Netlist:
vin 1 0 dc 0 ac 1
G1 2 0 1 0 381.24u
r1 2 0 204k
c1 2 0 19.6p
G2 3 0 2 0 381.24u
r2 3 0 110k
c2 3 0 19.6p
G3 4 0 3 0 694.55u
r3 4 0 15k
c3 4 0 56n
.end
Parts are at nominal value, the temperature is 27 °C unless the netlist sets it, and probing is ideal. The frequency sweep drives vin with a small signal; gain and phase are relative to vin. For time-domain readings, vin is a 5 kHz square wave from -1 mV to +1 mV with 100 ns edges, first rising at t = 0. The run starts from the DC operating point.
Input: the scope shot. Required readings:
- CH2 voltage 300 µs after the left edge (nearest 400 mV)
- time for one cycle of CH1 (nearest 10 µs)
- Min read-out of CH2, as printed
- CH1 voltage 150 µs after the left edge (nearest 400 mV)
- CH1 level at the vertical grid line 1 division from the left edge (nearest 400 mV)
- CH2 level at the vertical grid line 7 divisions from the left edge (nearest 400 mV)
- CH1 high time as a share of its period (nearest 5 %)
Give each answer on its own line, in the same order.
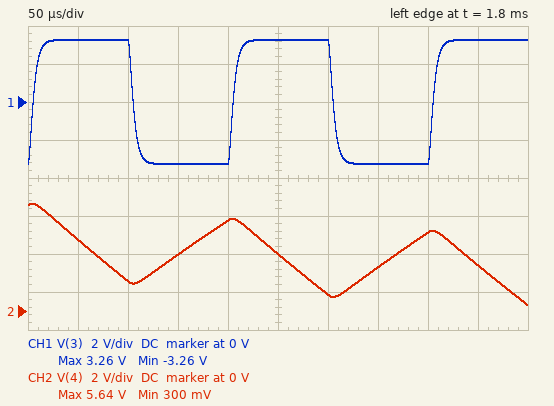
800 mV
200 µs
300 mV
-3.2 V
3.2 V
2.4 V
50 %
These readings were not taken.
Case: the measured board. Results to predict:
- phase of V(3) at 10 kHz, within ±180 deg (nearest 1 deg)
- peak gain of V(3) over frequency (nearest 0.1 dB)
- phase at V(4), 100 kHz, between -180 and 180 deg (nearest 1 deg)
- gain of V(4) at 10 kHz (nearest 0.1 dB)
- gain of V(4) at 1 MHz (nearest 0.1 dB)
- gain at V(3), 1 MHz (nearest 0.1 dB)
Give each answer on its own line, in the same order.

-22 deg
70.3 dB
-32 deg
55.8 dB
-34.5 dB
19.6 dB
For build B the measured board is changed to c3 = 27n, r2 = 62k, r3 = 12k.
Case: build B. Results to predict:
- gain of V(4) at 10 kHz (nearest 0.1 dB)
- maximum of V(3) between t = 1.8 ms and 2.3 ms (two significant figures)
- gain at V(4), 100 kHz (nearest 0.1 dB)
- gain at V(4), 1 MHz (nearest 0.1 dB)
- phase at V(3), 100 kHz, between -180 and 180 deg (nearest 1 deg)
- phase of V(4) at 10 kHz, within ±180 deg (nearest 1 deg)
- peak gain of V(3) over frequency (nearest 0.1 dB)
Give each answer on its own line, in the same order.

57.2 dB
1.8 V
26.9 dB
-28.2 dB
-106 deg
74 deg
65.3 dB
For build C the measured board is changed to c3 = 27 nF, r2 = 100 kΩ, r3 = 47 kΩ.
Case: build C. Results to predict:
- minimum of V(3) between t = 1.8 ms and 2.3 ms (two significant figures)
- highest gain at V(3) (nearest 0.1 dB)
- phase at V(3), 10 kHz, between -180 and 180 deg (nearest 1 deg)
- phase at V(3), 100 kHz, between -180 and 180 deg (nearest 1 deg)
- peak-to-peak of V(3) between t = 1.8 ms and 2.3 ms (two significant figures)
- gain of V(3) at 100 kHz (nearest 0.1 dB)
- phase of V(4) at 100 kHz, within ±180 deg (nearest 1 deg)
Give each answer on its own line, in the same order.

-3.0 V
69.4 dB
-21 deg
-119 deg
5.9 V
56.8 dB
-29 deg
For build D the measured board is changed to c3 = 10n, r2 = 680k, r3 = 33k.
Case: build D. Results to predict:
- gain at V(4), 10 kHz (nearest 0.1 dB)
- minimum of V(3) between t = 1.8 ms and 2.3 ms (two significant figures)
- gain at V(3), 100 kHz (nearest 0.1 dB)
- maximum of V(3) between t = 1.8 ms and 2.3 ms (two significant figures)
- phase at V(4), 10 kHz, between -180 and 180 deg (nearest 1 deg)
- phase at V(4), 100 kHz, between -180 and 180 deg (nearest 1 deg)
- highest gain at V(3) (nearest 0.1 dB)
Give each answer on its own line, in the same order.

84.4 dB
-20 V
58.9 dB
20 V
39 deg
-61 deg
86.1 dB
